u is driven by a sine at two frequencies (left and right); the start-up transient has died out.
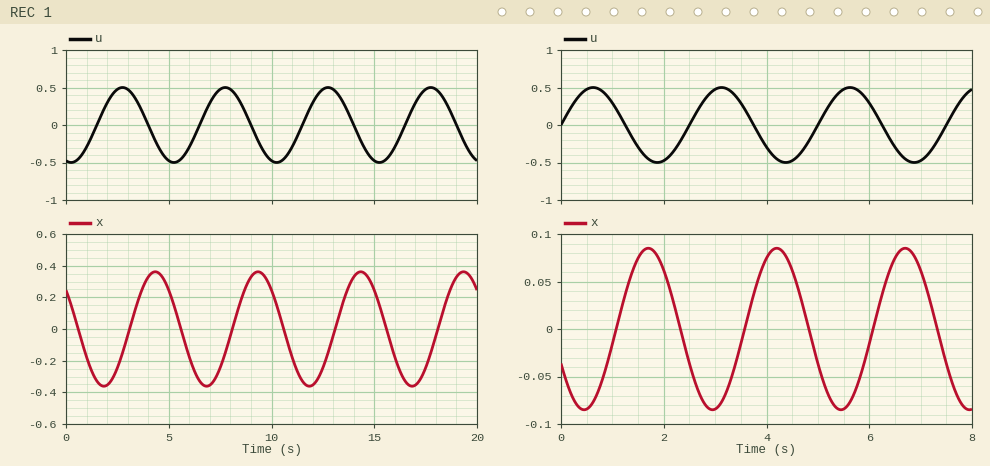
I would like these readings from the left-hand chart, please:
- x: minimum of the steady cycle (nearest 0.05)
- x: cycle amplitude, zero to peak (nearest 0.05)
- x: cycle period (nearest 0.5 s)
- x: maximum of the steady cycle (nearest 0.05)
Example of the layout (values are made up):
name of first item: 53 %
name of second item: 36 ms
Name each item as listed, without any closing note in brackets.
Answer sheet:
x: minimum of the steady cycle: -0.35
x: cycle amplitude, zero to peak: 0.35
x: cycle period: 5.0 s
x: maximum of the steady cycle: 0.35
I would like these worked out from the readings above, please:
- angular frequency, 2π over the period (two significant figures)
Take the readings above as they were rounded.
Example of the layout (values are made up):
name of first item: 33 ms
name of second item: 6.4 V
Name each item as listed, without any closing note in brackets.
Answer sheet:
angular frequency, 2π over the period: 1.3 rad/s
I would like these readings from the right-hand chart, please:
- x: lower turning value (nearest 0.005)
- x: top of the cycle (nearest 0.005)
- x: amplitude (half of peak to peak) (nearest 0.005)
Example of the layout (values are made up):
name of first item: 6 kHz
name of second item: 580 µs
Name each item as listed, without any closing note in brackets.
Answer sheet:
x: lower turning value: -0.085
x: top of the cycle: 0.085
x: amplitude (half of peak to peak): 0.085
